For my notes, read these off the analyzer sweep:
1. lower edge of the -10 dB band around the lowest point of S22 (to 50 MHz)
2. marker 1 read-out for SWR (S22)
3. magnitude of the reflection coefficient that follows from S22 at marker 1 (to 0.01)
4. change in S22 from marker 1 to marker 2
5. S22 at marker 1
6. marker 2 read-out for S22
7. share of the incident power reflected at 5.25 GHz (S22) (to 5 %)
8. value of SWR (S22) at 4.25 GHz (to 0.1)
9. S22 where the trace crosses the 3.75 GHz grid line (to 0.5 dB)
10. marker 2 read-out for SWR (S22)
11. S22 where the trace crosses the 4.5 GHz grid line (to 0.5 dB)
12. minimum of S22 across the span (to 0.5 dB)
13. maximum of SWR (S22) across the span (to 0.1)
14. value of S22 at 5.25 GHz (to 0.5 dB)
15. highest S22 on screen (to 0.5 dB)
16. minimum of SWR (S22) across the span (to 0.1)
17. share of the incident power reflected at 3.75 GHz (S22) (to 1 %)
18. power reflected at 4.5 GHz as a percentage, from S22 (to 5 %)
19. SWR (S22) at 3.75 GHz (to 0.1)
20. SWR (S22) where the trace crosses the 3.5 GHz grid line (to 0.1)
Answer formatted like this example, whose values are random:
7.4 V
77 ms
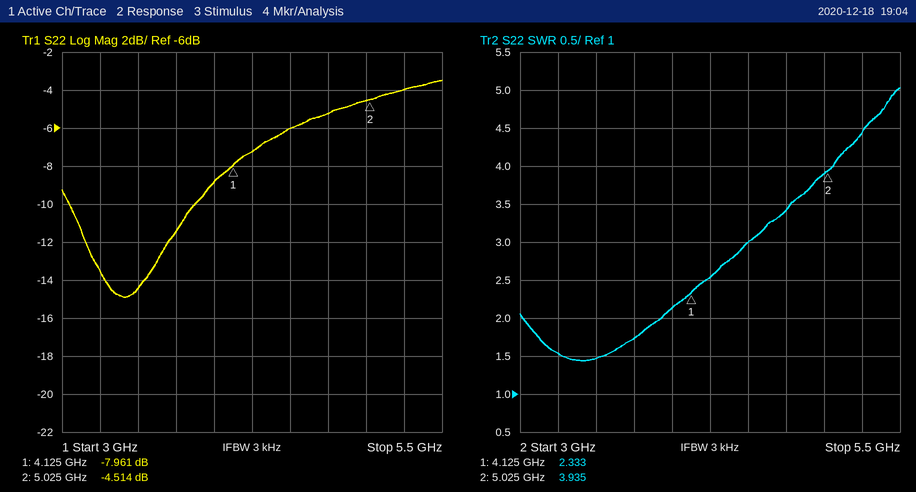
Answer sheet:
3.05 GHz
2.333
0.40
3.447 dB
-7.961 dB
-4.514 dB
40 %
2.5
-11.5 dB
3.935
-6.0 dB
-15.0 dB
5.0
-4.0 dB
-3.5 dB
1.4
7 %
25 %
1.7
1.5
